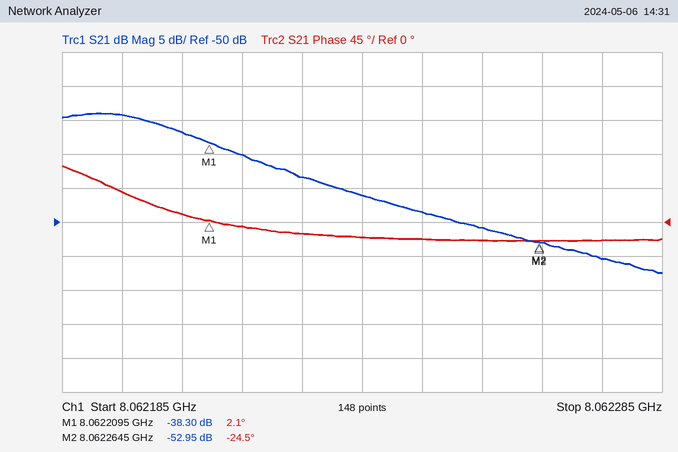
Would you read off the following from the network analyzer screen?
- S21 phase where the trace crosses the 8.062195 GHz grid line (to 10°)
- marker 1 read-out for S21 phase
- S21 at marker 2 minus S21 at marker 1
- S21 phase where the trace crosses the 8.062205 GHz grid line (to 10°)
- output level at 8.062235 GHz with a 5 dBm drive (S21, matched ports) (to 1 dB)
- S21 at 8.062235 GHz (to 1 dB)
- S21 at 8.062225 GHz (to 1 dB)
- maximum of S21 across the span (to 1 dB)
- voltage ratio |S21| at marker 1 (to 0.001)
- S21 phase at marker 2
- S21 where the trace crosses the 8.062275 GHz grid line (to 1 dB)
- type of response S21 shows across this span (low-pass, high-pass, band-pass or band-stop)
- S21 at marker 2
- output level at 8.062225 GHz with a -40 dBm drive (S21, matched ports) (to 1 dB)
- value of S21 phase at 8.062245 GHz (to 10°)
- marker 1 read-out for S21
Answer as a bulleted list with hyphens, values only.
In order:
- 40°
- 2.1°
- -14.65 dB
- 10°
- -41 dBm
- -46 dB
- -43 dB
- -34 dB
- 0.012
- -24.5°
- -55 dB
- low-pass
- -52.95 dB
- -83 dBm
- -20°
- -38.30 dB
